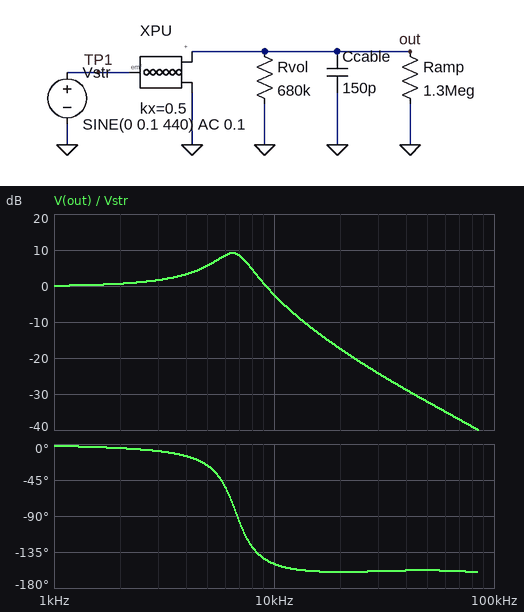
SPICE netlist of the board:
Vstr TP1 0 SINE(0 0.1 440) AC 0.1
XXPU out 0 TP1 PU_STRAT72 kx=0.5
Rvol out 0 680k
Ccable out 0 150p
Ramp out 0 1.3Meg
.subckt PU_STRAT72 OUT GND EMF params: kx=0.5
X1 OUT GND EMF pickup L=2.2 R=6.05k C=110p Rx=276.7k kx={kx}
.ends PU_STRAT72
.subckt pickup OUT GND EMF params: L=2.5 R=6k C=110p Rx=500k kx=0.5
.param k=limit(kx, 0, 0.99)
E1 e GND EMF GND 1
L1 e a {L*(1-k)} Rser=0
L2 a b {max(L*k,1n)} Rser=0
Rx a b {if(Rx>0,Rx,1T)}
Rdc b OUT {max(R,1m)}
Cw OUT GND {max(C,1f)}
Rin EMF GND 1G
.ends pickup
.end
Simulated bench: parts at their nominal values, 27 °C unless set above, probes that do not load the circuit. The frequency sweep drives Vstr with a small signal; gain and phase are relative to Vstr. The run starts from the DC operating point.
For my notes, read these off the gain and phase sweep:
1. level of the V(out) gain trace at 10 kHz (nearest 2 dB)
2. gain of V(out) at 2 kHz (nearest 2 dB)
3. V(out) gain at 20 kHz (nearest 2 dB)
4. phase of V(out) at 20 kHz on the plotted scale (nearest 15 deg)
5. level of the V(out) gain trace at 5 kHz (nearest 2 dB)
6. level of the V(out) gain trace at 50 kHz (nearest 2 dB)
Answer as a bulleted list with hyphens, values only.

- -2 dB
- 0 dB
- -18 dB
- -165 deg
- 6 dB
- -32 dB
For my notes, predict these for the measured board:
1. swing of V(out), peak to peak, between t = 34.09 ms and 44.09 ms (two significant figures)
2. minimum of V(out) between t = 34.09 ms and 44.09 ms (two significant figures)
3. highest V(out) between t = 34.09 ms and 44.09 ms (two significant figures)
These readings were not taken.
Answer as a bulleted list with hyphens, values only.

- 200 mV
- -99 mV
- 99 mV
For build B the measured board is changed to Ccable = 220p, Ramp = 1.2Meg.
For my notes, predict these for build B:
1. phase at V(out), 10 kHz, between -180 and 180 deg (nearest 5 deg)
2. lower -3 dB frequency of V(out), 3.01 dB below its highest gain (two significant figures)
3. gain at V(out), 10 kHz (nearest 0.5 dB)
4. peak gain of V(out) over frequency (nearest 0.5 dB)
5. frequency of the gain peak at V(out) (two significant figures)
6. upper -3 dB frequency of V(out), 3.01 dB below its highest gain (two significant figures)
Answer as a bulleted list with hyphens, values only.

- -155 deg
- 4.7 kHz
- -5.5 dB
- 9.5 dB
- 5.8 kHz
- 6.7 kHz
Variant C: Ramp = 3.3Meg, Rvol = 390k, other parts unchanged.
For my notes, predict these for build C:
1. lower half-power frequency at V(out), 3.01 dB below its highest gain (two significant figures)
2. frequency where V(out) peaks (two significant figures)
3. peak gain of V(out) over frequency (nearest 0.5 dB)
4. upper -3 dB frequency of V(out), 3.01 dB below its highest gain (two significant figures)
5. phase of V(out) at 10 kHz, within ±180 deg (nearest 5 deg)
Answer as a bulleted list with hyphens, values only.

- 4.8 kHz
- 6.4 kHz
- 8.0 dB
- 7.7 kHz
- -145 deg
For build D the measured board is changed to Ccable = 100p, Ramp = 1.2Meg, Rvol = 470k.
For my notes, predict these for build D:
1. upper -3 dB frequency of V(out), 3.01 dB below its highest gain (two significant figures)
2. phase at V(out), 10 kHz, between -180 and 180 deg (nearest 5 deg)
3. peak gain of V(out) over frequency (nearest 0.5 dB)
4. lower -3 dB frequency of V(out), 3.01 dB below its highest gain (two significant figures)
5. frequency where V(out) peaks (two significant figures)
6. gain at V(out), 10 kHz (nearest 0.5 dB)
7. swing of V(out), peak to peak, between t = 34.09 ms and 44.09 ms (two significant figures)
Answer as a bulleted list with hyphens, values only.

- 8.7 kHz
- -135 deg
- 7.0 dB
- 5.1 kHz
- 7.1 kHz
- 0 dB
- 200 mV
